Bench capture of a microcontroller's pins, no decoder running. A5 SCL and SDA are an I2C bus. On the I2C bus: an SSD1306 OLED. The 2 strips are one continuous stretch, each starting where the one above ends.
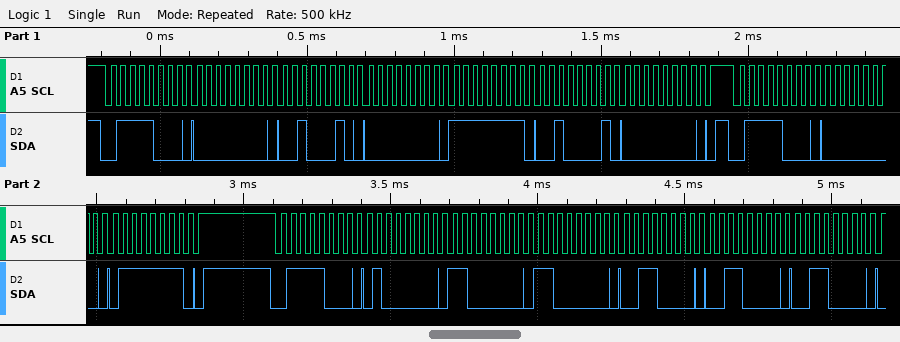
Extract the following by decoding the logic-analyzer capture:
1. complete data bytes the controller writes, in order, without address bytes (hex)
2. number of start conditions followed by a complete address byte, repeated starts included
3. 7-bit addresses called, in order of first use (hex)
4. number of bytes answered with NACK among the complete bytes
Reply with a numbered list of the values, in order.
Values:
1. 00 22 00 FF 21 00 00 7F 40 C0 C0 30 30 30
2. 3
3. 0x3C
4. 0
